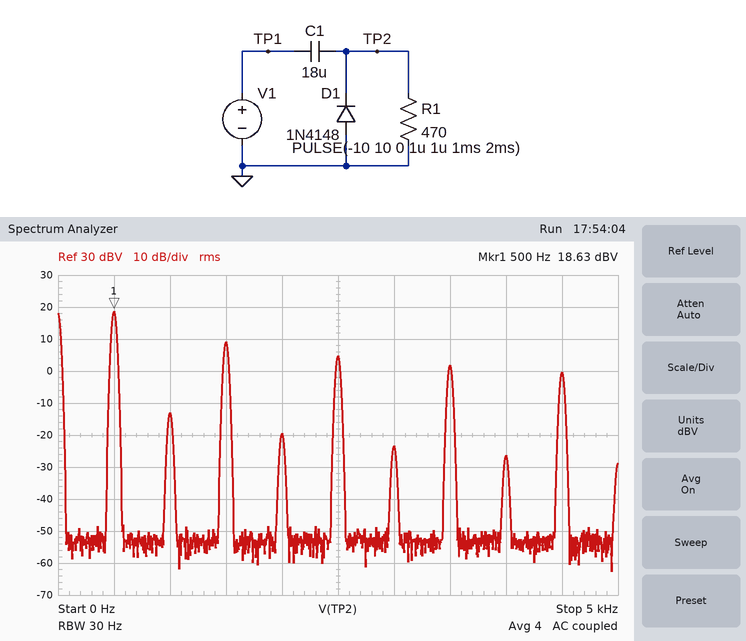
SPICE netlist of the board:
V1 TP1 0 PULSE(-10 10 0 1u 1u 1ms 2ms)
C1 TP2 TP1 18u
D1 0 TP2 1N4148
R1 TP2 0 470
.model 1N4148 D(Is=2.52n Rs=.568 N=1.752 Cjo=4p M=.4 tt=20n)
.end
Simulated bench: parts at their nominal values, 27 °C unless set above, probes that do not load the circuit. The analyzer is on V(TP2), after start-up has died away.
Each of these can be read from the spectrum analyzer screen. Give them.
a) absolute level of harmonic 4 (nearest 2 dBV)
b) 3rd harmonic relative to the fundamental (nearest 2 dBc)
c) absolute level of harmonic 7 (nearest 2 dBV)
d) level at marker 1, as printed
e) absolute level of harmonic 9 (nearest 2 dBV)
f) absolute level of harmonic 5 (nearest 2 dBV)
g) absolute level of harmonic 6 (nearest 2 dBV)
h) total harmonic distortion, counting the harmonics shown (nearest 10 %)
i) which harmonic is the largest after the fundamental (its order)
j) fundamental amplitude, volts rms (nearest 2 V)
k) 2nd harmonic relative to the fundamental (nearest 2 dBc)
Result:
-20 dBV
-10 dBc
2 dBV
18.63 dBV
0 dBV
4 dBV
-24 dBV
40 %
3
8 V
-32 dBc
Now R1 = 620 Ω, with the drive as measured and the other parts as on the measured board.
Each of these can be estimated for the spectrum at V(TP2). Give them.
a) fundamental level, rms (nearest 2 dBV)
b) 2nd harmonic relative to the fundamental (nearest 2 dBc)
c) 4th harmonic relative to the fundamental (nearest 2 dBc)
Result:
18 dBV
-34 dBc
-40 dBc
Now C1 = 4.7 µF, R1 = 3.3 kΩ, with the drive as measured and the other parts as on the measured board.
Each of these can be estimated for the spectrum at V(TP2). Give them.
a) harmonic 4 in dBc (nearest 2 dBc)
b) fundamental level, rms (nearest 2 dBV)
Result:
-44 dBc
18 dBV
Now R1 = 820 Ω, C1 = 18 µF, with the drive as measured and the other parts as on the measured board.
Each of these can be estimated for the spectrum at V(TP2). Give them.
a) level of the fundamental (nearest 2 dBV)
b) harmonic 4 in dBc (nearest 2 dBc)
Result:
18 dBV
-44 dBc
